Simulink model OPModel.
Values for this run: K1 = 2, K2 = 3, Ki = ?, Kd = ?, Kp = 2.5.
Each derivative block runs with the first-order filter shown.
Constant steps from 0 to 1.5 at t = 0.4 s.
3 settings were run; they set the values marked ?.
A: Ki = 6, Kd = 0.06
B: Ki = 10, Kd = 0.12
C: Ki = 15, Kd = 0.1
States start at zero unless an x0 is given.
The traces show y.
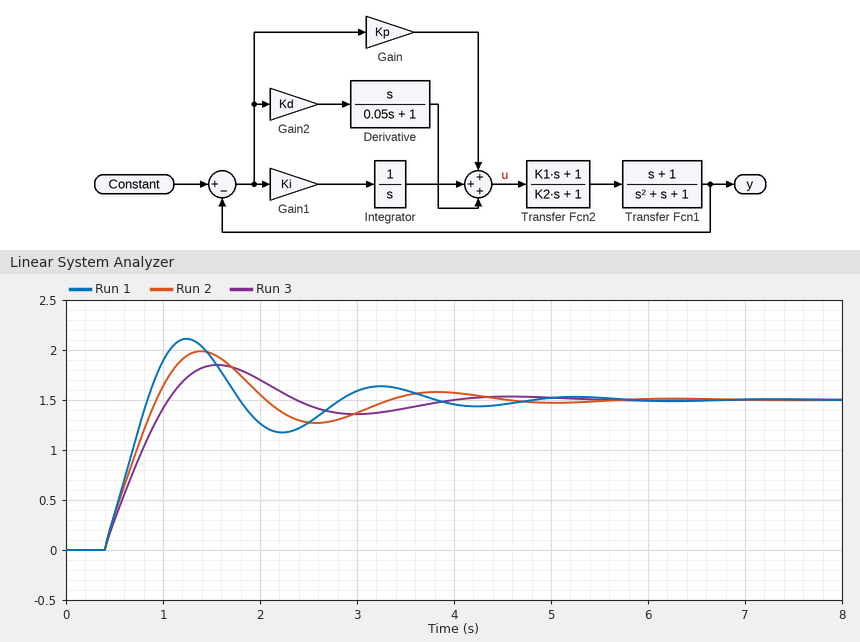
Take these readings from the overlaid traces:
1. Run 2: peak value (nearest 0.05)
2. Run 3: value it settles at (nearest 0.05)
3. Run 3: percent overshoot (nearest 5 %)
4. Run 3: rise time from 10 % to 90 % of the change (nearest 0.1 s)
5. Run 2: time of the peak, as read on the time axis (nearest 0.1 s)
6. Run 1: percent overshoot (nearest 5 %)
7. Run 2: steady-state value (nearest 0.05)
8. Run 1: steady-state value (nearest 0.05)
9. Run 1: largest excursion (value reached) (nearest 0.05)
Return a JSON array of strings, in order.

["2.00", "1.50", "25 %", "0.5 s", "1.4 s", "40 %", "1.50", "1.50", "2.10"]
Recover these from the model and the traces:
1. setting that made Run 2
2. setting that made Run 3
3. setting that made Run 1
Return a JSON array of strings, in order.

["B", "A", "C"]
